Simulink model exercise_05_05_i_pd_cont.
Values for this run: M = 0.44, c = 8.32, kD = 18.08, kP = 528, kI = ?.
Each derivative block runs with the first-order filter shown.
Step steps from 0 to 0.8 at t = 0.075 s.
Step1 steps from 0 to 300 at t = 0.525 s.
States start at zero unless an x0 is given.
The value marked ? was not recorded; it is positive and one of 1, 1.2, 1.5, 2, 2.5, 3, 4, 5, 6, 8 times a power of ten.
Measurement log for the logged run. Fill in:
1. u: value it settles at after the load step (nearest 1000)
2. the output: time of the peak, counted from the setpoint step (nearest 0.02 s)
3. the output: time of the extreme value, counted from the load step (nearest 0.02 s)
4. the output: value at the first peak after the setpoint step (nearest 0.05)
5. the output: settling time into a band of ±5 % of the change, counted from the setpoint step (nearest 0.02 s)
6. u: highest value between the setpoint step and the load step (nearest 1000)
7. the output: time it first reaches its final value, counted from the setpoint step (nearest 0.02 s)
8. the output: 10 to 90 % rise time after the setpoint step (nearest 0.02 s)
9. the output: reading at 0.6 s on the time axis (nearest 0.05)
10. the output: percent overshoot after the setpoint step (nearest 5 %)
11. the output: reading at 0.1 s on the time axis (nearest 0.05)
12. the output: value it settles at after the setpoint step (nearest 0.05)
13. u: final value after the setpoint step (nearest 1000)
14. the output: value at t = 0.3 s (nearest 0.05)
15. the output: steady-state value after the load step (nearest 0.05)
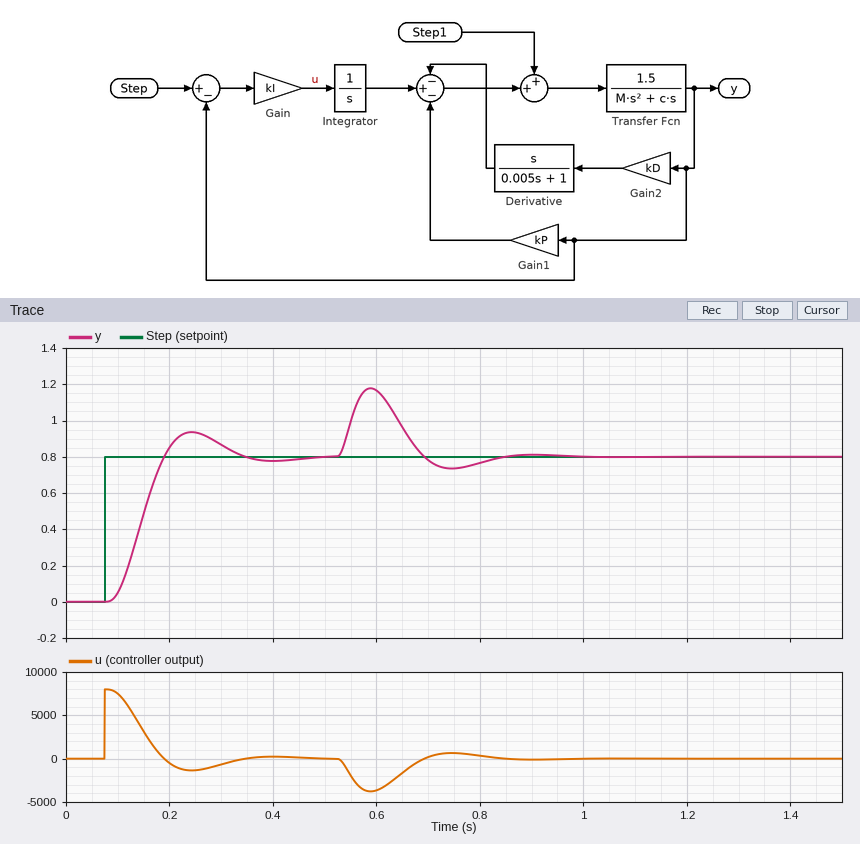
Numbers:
0
0.16 s
0.06 s
0.95
0.24 s
8000
0.12 s
0.08 s
1.15
15 %
0.05
0.80
0
0.85
0.80
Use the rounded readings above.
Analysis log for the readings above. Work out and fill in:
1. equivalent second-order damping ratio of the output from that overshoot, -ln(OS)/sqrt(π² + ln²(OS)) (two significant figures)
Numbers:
0.52
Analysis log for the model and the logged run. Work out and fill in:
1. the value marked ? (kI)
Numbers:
10000
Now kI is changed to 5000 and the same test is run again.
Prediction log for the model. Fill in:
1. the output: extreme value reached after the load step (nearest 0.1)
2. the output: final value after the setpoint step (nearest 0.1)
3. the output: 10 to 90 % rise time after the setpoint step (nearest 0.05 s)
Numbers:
1.2
0.8
0.15 s
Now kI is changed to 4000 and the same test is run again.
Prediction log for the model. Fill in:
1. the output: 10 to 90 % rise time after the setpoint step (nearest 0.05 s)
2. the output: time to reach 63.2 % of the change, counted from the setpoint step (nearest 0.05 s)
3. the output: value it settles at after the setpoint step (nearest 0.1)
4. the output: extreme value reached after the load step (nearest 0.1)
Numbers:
0.20 s
0.15 s
0.8
1.2
